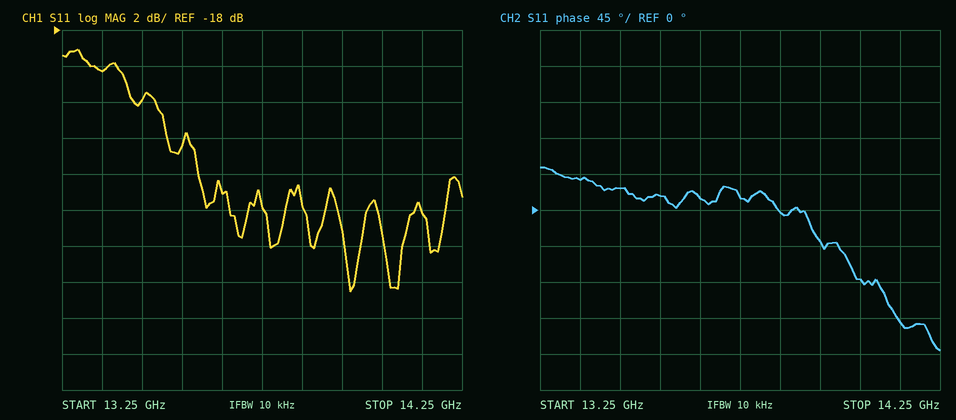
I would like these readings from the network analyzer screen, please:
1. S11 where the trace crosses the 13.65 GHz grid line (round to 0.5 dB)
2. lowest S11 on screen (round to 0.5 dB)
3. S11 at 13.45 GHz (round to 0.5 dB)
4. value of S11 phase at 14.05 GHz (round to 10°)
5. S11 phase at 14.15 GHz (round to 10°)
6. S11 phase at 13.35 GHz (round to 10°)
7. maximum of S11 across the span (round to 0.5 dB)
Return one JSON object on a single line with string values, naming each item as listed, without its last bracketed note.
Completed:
{"S11 where the trace crosses the 13.65 GHz grid line": "-27.0 dB", "lowest S11 on screen": "-32.5 dB", "S11 at 13.45 GHz": "-22.0 dB", "value of S11 phase at 14.05 GHz": "-90°", "S11 phase at 14.15 GHz": "-140°", "S11 phase at 13.35 GHz": "40°", "maximum of S11 across the span": "-19.0 dB"}
